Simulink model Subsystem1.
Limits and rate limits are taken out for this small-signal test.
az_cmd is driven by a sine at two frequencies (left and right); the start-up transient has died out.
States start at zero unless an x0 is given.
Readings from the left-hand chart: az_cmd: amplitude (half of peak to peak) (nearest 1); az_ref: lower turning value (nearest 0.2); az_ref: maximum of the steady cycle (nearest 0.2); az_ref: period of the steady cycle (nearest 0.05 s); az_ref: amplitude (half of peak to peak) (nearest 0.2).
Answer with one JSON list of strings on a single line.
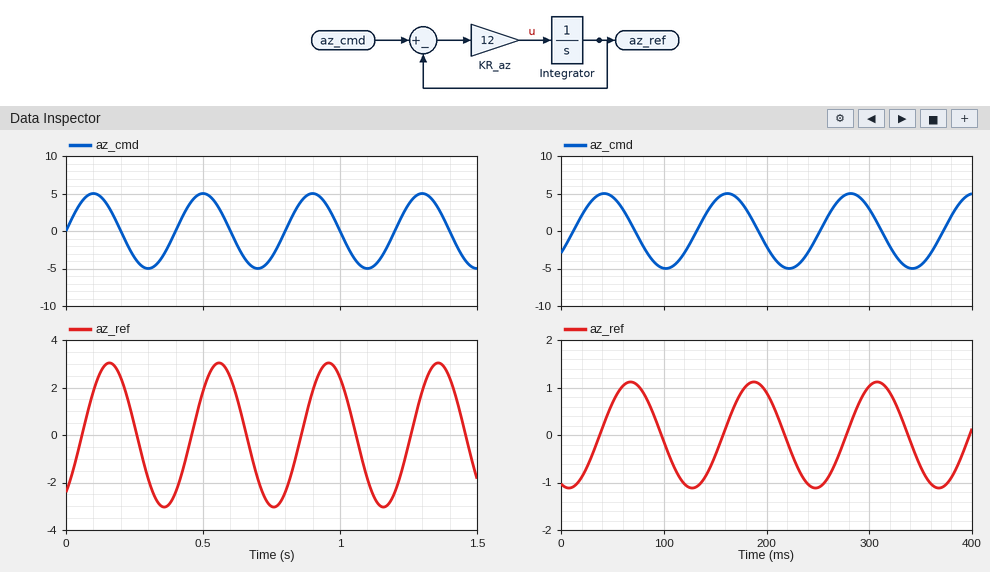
["5", "-3.0", "3.0", "0.40 s", "3.0"]
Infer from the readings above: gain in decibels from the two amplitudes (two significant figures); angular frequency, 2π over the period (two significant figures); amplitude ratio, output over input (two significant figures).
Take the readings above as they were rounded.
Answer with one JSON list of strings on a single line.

["-4.4 dB", "16 rad/s", "0.60"]
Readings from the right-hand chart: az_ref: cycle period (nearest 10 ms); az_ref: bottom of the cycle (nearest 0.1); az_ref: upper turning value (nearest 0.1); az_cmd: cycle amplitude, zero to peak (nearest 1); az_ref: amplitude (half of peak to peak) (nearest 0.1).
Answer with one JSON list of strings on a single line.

["120 ms", "-1.1", "1.1", "5", "1.1"]
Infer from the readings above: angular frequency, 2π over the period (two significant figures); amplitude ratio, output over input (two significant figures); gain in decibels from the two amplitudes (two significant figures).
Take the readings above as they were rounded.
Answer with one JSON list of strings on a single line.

["0.052 rad/ms", "0.22", "-13 dB"]
